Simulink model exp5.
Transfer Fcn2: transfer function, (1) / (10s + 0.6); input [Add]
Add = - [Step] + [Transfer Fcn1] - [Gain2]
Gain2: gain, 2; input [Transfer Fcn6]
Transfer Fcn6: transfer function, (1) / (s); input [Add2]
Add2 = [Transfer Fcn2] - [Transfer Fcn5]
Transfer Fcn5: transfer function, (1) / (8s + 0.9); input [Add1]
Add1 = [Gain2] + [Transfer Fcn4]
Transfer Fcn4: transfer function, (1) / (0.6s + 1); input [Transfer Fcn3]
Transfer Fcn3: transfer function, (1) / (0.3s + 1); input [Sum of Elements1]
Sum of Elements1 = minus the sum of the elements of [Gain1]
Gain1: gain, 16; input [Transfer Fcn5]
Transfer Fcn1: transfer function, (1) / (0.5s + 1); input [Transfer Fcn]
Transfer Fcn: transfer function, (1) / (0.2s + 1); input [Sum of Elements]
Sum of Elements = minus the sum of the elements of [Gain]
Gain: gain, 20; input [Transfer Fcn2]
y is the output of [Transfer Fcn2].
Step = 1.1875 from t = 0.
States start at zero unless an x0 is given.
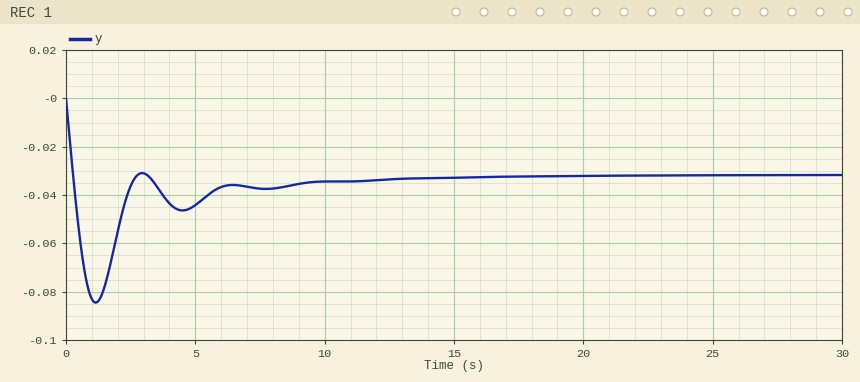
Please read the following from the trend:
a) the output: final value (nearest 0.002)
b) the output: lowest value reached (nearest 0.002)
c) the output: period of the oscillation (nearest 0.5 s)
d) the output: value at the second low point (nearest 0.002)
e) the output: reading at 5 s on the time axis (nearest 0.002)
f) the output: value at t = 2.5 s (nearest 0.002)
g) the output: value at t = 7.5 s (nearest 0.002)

-0.032
-0.084
3.5 s
-0.046
-0.044
-0.036
-0.038
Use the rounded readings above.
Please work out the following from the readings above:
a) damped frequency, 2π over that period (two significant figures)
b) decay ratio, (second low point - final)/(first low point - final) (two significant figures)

1.8 rad/s
0.27
